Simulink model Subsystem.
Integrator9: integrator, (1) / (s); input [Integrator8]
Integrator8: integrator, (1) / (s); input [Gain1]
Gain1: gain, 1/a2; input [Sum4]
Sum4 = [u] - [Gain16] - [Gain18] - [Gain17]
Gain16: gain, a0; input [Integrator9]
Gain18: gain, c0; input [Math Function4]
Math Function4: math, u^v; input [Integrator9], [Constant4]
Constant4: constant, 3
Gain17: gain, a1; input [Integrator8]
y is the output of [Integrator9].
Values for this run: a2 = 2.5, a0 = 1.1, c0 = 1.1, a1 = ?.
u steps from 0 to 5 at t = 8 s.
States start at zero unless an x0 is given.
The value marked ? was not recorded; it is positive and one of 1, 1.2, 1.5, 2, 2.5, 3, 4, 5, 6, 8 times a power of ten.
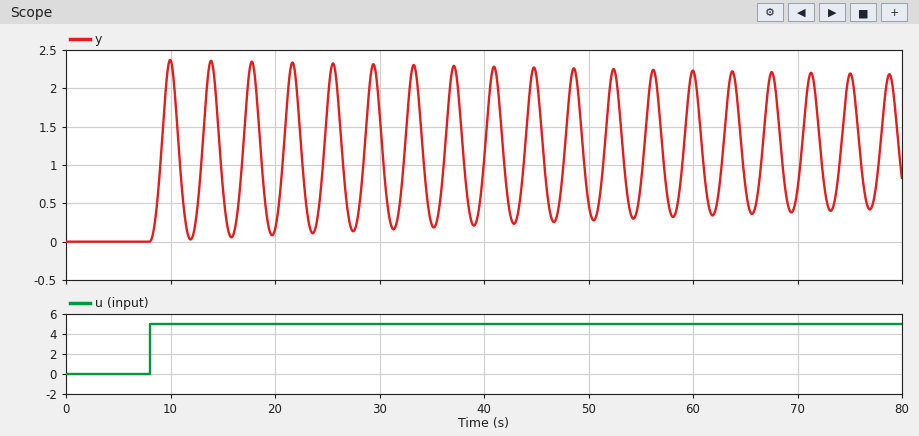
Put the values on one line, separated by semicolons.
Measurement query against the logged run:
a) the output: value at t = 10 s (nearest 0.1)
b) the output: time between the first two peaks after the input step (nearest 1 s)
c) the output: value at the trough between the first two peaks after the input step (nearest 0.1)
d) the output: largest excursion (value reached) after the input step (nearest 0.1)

2.4; 4 s; 0.0; 2.4
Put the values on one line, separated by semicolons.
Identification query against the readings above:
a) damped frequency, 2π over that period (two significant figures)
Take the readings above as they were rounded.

1.6 rad/s
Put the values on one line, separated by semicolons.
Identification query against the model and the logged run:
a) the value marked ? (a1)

0.02
